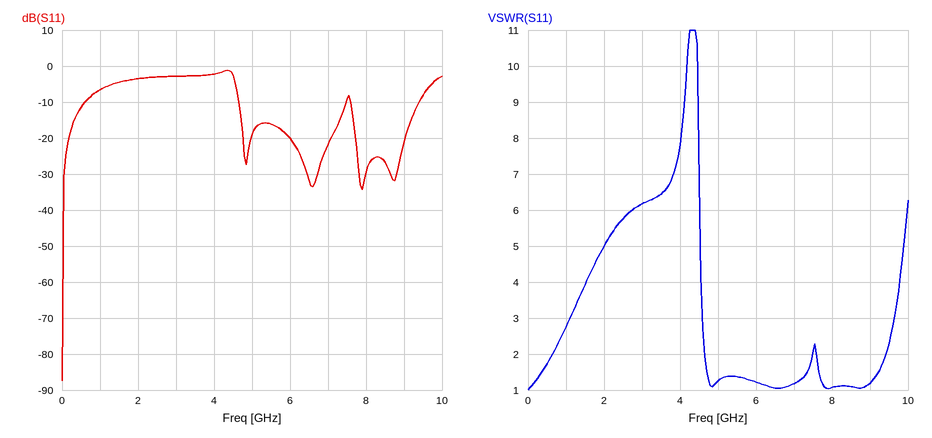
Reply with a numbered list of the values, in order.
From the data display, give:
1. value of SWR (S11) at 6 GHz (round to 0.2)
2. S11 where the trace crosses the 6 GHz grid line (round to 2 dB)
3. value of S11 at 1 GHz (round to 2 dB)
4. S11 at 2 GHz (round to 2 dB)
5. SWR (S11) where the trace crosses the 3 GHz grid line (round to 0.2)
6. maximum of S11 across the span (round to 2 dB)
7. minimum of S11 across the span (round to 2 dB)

1. 1.2
2. -20 dB
3. -6 dB
4. -4 dB
5. 6.2
6. -2 dB
7. -88 dB
